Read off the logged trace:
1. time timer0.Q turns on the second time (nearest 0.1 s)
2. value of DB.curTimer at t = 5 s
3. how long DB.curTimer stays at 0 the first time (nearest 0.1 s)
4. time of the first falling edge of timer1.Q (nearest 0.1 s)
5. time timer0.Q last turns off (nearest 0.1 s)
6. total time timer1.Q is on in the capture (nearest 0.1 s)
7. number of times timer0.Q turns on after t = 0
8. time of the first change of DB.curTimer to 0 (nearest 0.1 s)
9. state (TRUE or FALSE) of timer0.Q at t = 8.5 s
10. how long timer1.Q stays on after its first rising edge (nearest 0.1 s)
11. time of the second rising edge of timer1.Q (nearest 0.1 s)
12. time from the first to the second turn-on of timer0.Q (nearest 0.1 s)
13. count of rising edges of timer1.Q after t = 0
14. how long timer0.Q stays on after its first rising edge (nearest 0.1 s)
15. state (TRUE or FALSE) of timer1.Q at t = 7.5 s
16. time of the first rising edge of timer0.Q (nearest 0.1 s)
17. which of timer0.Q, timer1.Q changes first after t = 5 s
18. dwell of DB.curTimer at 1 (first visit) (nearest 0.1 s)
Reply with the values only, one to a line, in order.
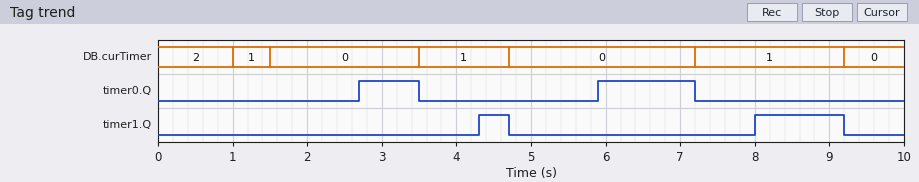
5.9 s
0
2.0 s
4.7 s
7.2 s
1.6 s
2
1.5 s
FALSE
0.4 s
8.0 s
3.2 s
2
0.8 s
FALSE
2.7 s
timer0.Q
0.5 s
